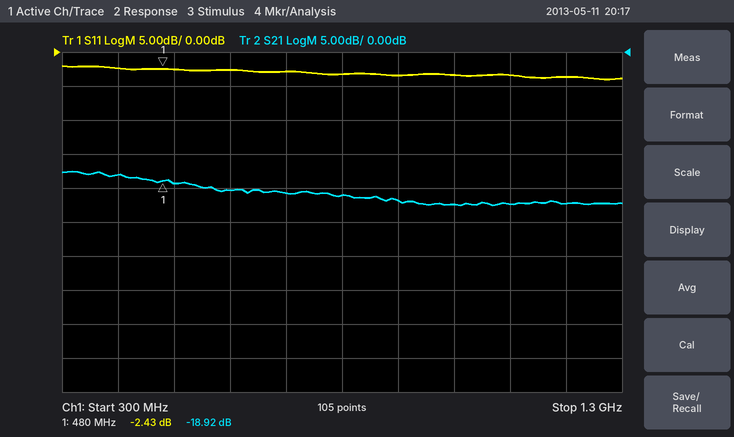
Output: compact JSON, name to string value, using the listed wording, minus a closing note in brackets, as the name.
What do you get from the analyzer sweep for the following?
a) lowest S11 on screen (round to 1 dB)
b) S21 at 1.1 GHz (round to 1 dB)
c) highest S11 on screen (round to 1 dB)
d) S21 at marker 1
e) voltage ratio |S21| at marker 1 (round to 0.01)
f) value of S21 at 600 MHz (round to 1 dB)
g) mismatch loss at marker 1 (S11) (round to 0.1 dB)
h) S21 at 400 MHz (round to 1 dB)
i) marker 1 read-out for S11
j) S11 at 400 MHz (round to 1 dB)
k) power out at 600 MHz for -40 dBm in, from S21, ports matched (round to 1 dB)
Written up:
{"lowest S11 on screen": "-4 dB", "S21 at 1.1 GHz": "-22 dB", "highest S11 on screen": "-2 dB", "S21 at marker 1": "-18.92 dB", "voltage ratio |S21| at marker 1": "0.11", "value of S21 at 600 MHz": "-20 dB", "mismatch loss at marker 1 (S11)": "3.7 dB", "S21 at 400 MHz": "-18 dB", "marker 1 read-out for S11": "-2.43 dB", "S11 at 400 MHz": "-2 dB", "power out at 600 MHz for -40 dBm in, from S21, ports matched": "-60 dBm"}
